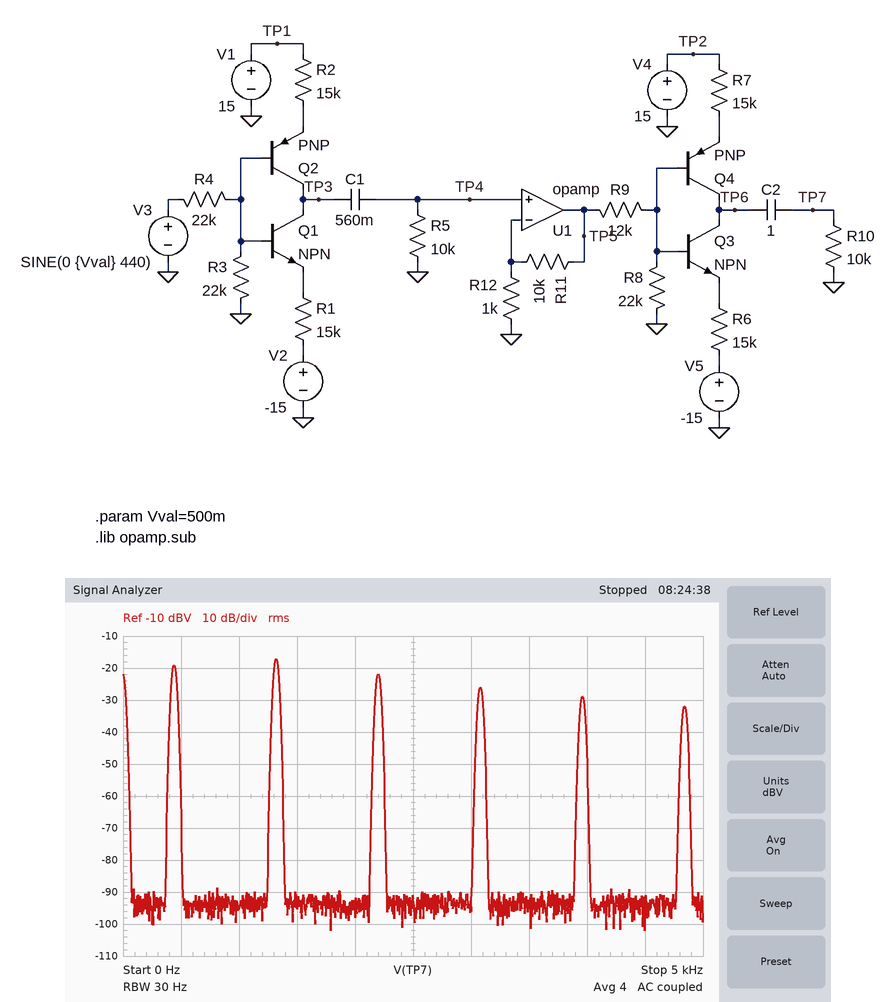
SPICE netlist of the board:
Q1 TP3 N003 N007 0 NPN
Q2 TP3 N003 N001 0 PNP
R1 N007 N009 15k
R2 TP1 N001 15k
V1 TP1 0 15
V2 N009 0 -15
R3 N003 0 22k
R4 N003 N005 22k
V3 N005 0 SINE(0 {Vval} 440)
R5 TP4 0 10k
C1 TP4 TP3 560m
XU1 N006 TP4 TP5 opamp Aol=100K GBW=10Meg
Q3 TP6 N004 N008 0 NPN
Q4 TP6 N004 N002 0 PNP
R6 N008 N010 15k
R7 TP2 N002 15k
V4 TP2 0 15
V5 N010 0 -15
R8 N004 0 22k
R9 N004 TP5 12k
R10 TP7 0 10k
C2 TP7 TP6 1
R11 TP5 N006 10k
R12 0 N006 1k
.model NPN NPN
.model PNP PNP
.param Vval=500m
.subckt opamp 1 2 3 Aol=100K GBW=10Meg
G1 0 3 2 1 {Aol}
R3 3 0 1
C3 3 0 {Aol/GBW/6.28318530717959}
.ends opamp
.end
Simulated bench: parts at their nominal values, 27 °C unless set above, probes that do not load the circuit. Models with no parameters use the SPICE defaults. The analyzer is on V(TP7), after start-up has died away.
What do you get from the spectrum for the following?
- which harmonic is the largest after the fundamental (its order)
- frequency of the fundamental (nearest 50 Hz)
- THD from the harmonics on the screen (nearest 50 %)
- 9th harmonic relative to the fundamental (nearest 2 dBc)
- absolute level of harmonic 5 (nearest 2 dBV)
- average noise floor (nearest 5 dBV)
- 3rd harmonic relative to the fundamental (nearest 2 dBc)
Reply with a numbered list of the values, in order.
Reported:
1. 3
2. 450 Hz
3. 150 %
4. -10 dBc
5. -22 dBV
6. -95 dBV
7. 2 dBc
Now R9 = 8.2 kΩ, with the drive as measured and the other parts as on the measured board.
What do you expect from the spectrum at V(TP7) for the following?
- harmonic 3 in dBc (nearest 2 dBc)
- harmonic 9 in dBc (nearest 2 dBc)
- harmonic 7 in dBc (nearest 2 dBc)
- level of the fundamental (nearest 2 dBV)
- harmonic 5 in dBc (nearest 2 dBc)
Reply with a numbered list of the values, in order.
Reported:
1. -6 dBc
2. -16 dBc
3. -14 dBc
4. -12 dBV
5. -10 dBc
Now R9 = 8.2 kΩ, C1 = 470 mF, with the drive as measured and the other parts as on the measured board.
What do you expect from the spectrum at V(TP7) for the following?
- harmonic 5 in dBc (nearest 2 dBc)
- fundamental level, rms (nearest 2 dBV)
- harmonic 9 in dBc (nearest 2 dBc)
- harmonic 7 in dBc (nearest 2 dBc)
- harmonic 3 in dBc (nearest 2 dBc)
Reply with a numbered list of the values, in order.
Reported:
1. -10 dBc
2. -12 dBV
3. -16 dBc
4. -14 dBc
5. -6 dBc
